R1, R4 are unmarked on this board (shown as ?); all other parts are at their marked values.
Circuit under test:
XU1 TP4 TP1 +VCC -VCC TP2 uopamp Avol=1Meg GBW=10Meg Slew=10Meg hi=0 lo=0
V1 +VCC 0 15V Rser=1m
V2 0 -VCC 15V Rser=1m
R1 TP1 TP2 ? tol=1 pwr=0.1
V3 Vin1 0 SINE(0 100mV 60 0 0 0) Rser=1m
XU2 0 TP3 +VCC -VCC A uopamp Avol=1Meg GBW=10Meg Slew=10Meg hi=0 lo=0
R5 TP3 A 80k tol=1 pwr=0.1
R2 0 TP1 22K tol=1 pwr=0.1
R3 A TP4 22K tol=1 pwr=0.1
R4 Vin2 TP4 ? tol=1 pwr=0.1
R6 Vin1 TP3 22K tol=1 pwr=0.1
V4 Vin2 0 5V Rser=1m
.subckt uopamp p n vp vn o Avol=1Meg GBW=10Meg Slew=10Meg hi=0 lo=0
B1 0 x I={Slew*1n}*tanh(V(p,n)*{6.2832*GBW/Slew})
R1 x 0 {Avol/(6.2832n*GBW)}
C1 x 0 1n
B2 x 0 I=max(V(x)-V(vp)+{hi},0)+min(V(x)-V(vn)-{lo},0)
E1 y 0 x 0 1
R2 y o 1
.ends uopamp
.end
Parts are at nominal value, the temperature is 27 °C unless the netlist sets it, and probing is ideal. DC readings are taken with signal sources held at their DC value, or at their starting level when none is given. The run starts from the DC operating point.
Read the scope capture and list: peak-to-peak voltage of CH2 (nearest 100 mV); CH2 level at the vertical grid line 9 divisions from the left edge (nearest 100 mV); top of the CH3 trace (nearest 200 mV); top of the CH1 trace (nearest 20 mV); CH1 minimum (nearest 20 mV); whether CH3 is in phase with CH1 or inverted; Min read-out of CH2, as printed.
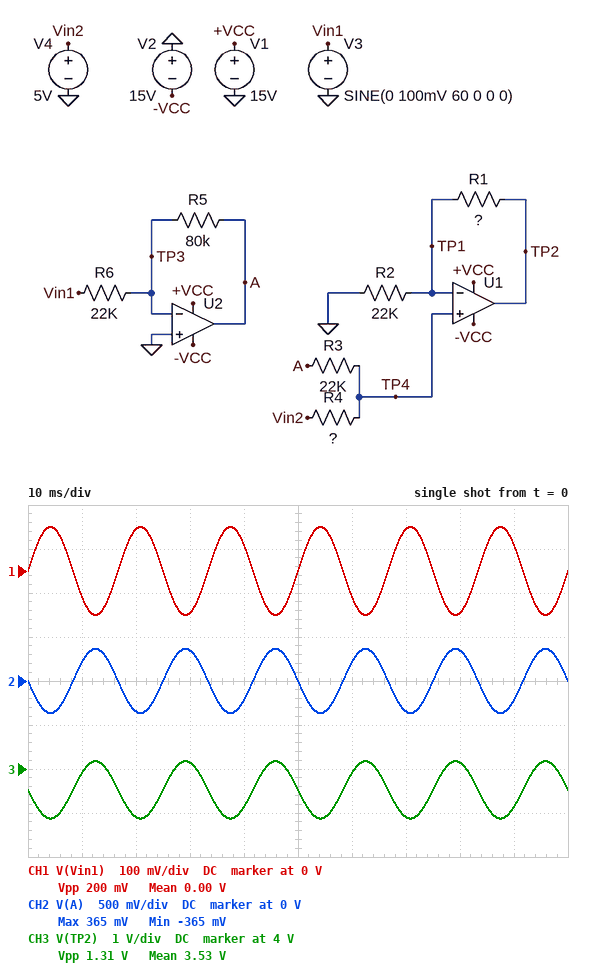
700 mV
-200 mV
4.2 V
100 mV
-100 mV
inverted
-365 mV
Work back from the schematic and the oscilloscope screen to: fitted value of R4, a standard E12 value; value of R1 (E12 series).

56 kΩ
33 kΩ
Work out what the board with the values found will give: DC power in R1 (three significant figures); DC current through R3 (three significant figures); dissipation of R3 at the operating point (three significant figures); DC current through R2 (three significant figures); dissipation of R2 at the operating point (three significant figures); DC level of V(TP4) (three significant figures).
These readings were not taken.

136 µW
64.1 µA
90.4 µW
64.1 µA
90.4 µW
1.41 V
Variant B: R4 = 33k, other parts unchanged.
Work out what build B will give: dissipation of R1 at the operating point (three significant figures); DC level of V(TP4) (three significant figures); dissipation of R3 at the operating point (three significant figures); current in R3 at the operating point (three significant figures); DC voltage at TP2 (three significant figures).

273 µW
2.00 V
182 µW
90.9 µA
5.00 V
